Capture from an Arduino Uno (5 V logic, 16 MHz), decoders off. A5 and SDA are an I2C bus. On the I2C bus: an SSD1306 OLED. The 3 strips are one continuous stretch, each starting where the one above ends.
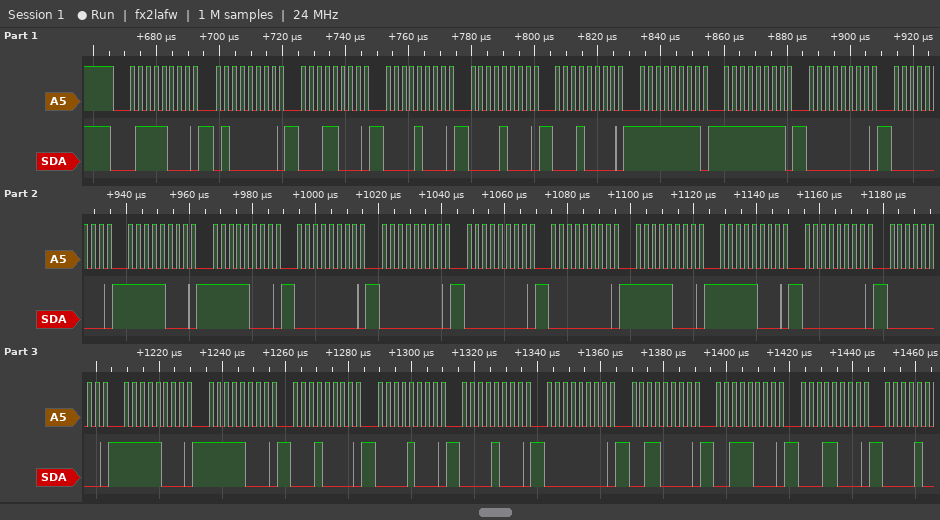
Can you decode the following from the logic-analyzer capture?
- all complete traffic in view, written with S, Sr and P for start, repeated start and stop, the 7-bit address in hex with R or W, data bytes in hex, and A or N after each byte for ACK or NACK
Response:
S 3CW A 40 A 18 A 08 A 08 A 10 A FF A FF A 00 A 00 A F8 A F8 A 00 A 00 A 00 A 00 A F8 A F8 A 00 A 00 A F8 A F8 A 10 A 08 A 08 A 00 A 30 A 38 A 18 A
